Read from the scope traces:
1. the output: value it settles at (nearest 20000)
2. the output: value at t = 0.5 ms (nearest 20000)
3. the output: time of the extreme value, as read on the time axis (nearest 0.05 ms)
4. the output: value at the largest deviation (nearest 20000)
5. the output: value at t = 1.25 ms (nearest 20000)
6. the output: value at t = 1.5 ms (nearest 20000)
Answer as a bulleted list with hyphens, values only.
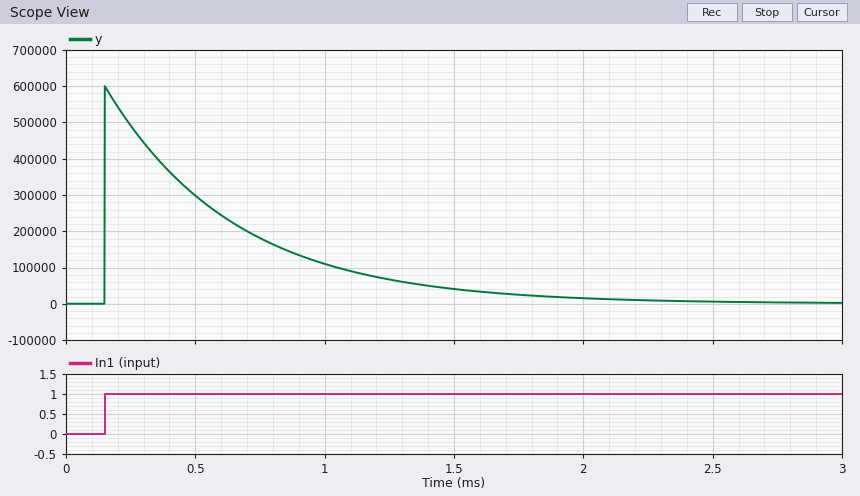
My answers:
- 0
- 300000
- 0.15 ms
- 600000
- 60000
- 40000
